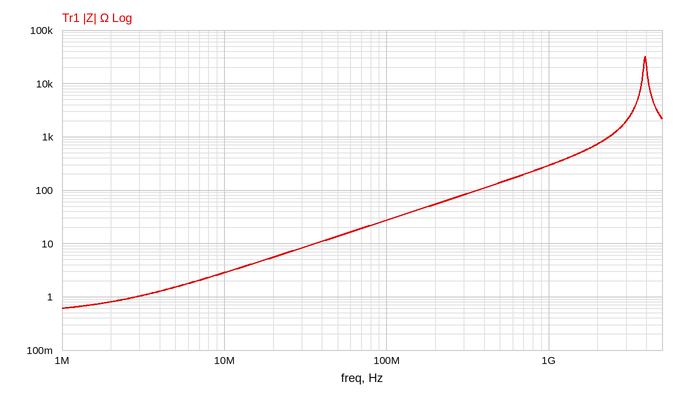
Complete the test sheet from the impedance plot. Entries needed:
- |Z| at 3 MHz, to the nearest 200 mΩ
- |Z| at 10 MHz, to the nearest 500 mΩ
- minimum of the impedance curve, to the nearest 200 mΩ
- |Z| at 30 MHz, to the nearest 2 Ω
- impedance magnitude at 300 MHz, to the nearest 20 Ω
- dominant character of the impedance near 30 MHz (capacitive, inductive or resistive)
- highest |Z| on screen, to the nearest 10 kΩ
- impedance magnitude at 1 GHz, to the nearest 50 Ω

1.0 Ω
3.0 Ω
600 mΩ
8 Ω
80 Ω
inductive
30 kΩ
300 Ω
